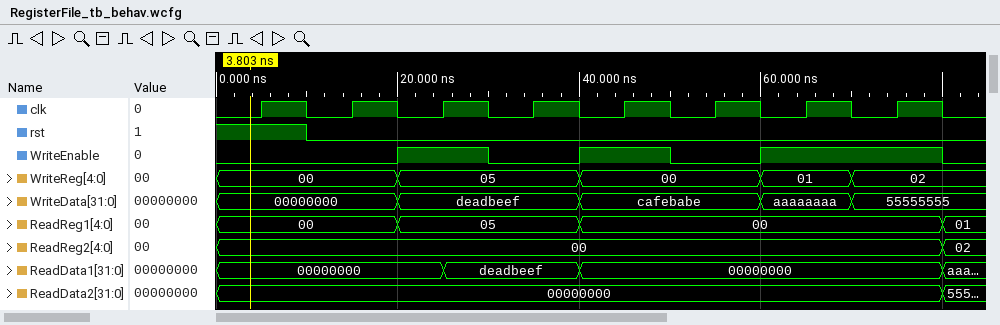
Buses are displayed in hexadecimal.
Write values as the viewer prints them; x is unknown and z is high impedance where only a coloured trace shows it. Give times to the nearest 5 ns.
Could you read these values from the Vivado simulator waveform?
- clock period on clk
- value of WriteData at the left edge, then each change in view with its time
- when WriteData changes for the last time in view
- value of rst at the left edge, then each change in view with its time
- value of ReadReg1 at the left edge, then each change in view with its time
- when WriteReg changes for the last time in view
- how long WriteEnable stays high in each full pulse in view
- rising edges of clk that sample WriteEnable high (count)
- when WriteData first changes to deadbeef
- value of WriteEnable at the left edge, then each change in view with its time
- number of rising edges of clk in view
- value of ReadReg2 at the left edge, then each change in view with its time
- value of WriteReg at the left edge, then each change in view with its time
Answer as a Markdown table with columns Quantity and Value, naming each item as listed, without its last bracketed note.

| Quantity | Value |
|---|---|
| clock period on clk | 10 ns |
| value of WriteData at the left edge, then each change in view with its time | 00000000, deadbeef at 20 ns, cafebabe at 40 ns, aaaaaaaa at 60 ns, 55555555 at 70 ns |
| when WriteData changes for the last time in view | 70 ns |
| value of rst at the left edge, then each change in view with its time | 1, 0 at 10 ns |
| value of ReadReg1 at the left edge, then each change in view with its time | 00, 05 at 20 ns, 00 at 40 ns, 01 at 80 ns |
| when WriteReg changes for the last time in view | 70 ns |
| how long WriteEnable stays high in each full pulse in view | 10 ns, 10 ns, 20 ns |
| rising edges of clk that sample WriteEnable high | 4 |
| when WriteData first changes to deadbeef | 20 ns |
| value of WriteEnable at the left edge, then each change in view with its time | 0, 1 at 20 ns, 0 at 30 ns, 1 at 40 ns, 0 at 50 ns, 1 at 60 ns, 0 at 80 ns |
| number of rising edges of clk in view | 8 |
| value of ReadReg2 at the left edge, then each change in view with its time | 00, 02 at 80 ns |
| value of WriteReg at the left edge, then each change in view with its time | 00, 05 at 20 ns, 00 at 40 ns, 01 at 60 ns, 02 at 70 ns |
